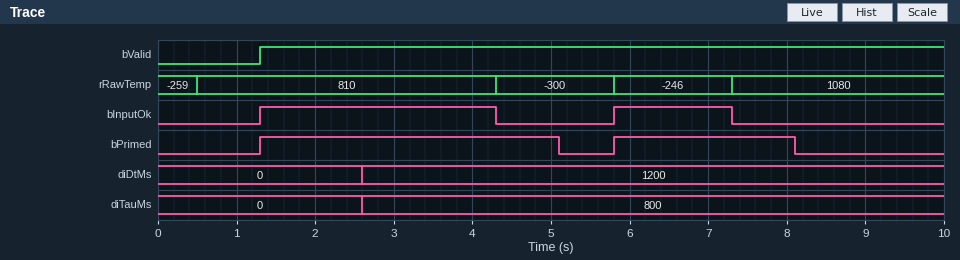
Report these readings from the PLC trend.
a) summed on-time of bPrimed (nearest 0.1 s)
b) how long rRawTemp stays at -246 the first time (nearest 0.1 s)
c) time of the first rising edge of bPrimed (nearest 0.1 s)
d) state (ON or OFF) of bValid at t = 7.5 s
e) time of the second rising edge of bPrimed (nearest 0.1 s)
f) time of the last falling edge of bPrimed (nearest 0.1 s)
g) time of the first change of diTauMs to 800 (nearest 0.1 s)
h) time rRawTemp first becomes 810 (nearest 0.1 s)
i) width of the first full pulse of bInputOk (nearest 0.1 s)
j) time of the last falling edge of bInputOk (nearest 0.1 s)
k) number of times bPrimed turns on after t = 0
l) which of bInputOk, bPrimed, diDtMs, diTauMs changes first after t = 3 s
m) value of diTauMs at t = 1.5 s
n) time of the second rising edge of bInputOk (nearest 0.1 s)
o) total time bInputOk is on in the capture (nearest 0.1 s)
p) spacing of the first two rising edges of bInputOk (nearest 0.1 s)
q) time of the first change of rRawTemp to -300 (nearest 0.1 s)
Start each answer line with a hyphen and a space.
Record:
- 6.1 s
- 1.5 s
- 1.3 s
- ON
- 5.8 s
- 8.1 s
- 2.6 s
- 0.5 s
- 3.0 s
- 7.3 s
- 2
- bInputOk
- 0
- 5.8 s
- 4.5 s
- 4.5 s
- 4.3 s
